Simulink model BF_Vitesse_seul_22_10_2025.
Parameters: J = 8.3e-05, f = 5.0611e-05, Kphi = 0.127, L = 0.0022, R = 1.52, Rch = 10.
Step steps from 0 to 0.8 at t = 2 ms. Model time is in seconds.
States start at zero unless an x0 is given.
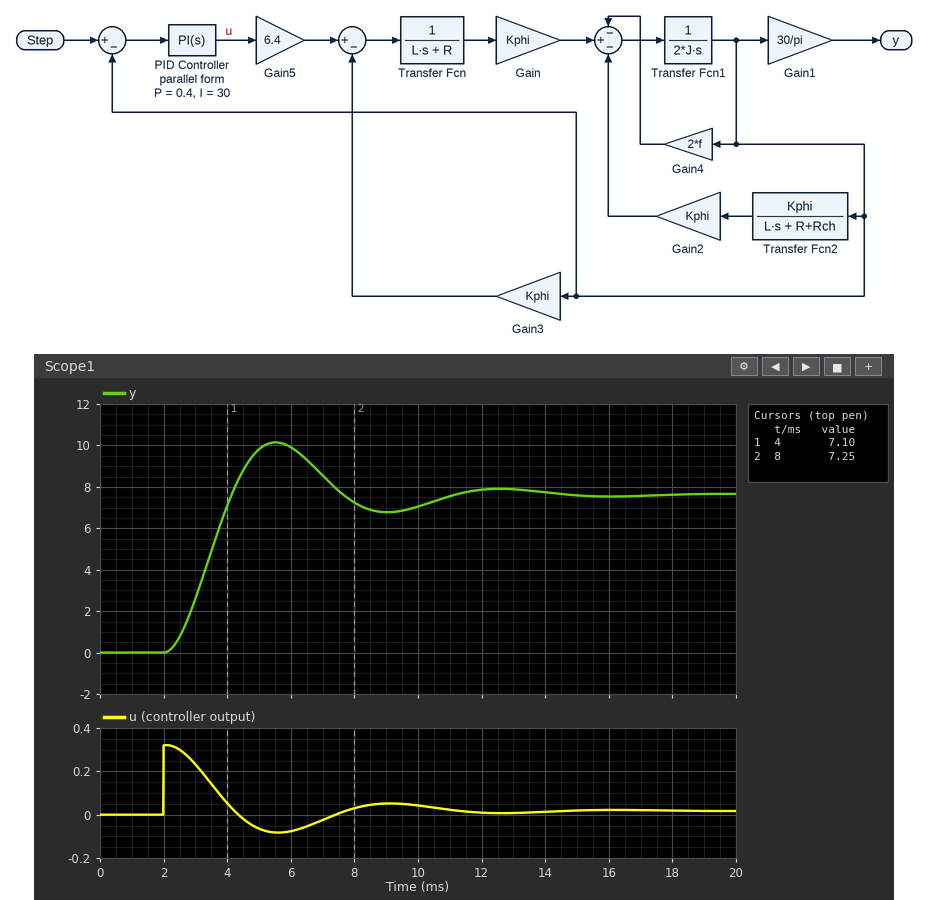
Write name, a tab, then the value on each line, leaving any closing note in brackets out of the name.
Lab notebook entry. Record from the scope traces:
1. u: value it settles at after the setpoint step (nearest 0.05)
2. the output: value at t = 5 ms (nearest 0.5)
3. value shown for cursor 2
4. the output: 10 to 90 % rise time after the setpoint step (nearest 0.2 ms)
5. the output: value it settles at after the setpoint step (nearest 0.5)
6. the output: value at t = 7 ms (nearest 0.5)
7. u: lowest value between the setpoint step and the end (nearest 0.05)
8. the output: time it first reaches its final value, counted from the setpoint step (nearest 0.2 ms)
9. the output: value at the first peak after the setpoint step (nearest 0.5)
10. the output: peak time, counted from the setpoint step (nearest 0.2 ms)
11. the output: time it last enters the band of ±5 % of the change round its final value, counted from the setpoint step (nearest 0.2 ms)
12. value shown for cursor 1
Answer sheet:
u: value it settles at after the setpoint step	0.00
the output: value at t = 5 ms	10.0
value shown for cursor 2	7.25
the output: 10 to 90 % rise time after the setpoint step	1.4 ms
the output: value it settles at after the setpoint step	7.5
the output: value at t = 7 ms	8.5
u: lowest value between the setpoint step and the end	-0.10
the output: time it first reaches its final value, counted from the setpoint step	2.2 ms
the output: value at the first peak after the setpoint step	10.0
the output: peak time, counted from the setpoint step	3.6 ms
the output: time it last enters the band of ±5 % of the change round its final value, counted from the setpoint step	8.4 ms
value shown for cursor 1	7.10
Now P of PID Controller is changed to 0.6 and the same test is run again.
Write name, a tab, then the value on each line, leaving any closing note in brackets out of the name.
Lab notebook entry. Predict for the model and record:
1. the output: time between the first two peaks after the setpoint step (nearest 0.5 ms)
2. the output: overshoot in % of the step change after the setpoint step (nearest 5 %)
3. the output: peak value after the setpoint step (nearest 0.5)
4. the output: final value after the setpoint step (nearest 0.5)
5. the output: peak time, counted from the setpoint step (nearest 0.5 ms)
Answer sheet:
the output: time between the first two peaks after the setpoint step	5.5 ms
the output: overshoot in % of the step change after the setpoint step	40 %
the output: peak value after the setpoint step	10.5
the output: final value after the setpoint step	7.5
the output: peak time, counted from the setpoint step	3.0 ms
